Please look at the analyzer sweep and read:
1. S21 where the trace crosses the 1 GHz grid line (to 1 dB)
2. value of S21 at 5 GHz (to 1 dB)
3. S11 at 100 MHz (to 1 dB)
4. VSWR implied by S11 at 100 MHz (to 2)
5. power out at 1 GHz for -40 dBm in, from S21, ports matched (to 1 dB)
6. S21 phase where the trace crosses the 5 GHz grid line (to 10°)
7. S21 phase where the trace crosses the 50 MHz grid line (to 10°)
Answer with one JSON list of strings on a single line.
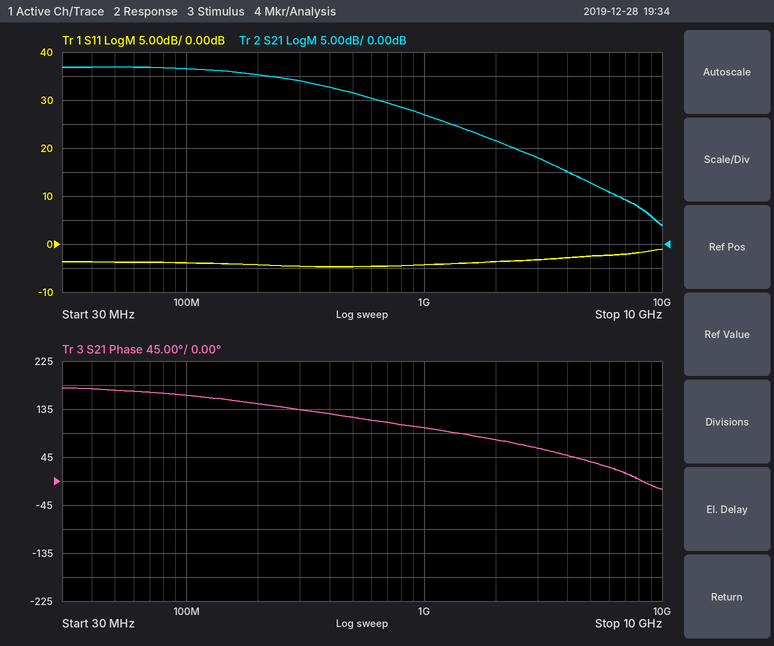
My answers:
["27 dB", "13 dB", "-4 dB", "4", "-13 dBm", "40°", "170°"]
